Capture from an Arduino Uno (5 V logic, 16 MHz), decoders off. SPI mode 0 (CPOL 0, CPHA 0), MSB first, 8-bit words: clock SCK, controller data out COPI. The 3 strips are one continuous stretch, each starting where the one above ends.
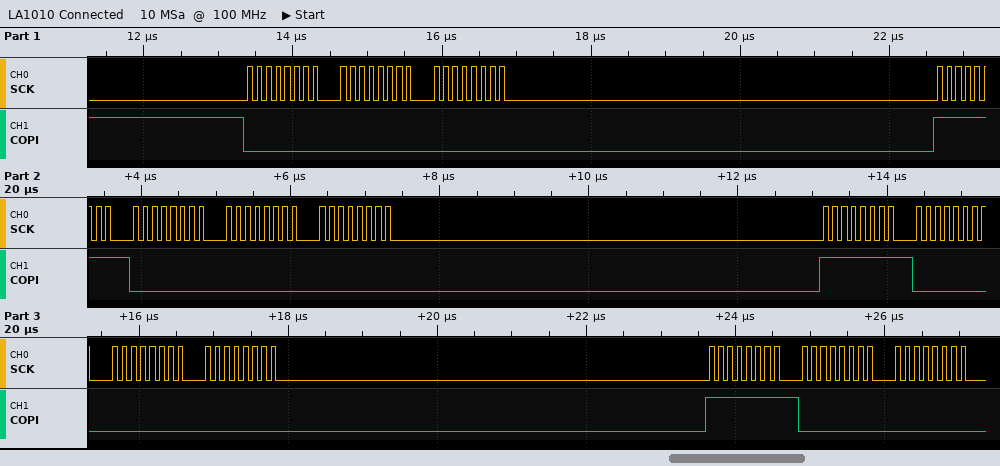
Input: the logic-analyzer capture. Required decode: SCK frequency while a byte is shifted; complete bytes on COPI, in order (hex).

8 MHz
0x00 0x00 0x00 0xFF 0x00 0x00 0x00 0xFF 0x00 0x00 0x00 0xFF 0x00 0x00
